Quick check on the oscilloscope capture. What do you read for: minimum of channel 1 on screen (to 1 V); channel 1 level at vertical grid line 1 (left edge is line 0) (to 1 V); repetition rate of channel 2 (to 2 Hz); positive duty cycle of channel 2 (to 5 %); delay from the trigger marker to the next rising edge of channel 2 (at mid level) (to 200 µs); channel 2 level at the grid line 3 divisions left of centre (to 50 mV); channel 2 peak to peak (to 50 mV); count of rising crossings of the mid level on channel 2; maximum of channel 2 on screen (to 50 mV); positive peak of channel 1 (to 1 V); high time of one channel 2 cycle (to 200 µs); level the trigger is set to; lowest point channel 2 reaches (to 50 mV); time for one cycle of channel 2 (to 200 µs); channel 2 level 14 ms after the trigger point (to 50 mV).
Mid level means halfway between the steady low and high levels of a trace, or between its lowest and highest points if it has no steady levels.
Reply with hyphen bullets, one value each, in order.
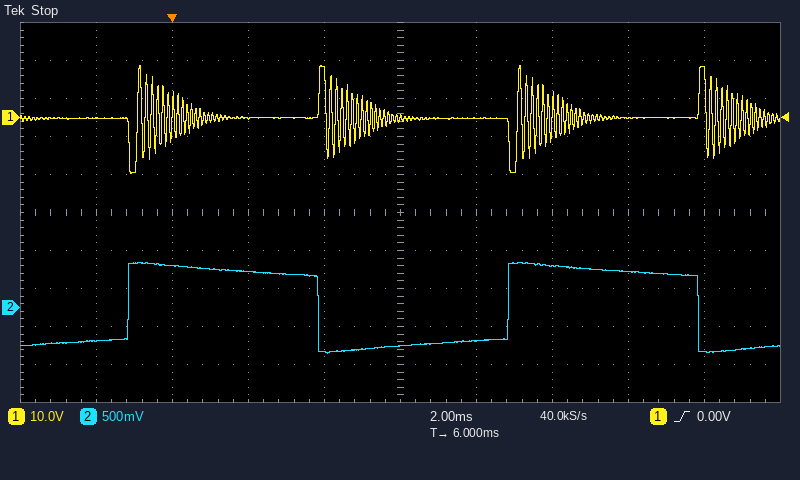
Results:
- -15 V
- 0 V
- 100 Hz
- 50 %
- 8.8 ms
- 550 mV
- 1.20 V
- 2
- 600 mV
- 14 V
- 5.0 ms
- 0.00 V
- -600 mV
- 10.0 ms
- -600 mV
